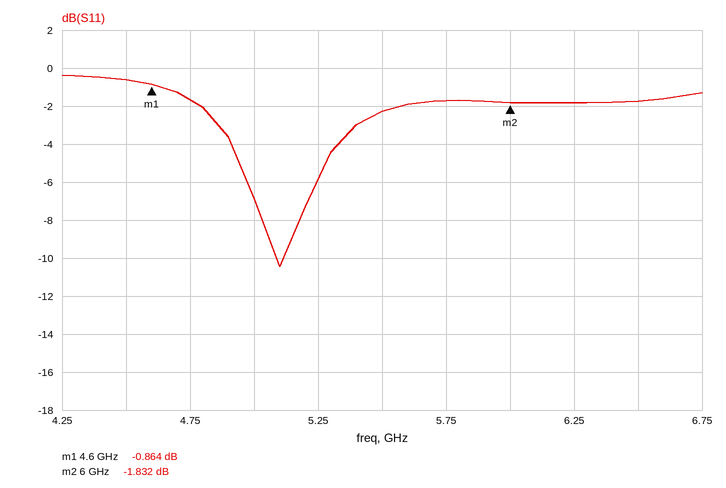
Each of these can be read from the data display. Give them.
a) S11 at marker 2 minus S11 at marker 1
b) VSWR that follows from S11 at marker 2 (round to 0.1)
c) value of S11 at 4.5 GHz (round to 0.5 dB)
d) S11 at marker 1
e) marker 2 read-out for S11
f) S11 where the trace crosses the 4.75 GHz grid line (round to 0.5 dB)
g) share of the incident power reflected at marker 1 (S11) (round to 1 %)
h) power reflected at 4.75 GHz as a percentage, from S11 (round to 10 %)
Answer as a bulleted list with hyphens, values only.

- -0.968 dB
- 9.5
- -0.5 dB
- -0.864 dB
- -1.832 dB
- -1.5 dB
- 82 %
- 70 %
